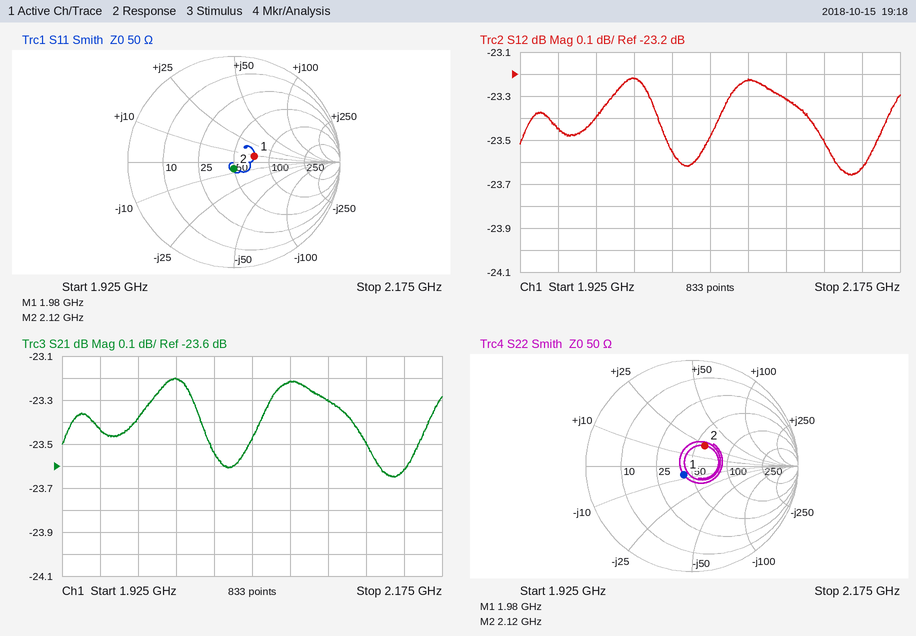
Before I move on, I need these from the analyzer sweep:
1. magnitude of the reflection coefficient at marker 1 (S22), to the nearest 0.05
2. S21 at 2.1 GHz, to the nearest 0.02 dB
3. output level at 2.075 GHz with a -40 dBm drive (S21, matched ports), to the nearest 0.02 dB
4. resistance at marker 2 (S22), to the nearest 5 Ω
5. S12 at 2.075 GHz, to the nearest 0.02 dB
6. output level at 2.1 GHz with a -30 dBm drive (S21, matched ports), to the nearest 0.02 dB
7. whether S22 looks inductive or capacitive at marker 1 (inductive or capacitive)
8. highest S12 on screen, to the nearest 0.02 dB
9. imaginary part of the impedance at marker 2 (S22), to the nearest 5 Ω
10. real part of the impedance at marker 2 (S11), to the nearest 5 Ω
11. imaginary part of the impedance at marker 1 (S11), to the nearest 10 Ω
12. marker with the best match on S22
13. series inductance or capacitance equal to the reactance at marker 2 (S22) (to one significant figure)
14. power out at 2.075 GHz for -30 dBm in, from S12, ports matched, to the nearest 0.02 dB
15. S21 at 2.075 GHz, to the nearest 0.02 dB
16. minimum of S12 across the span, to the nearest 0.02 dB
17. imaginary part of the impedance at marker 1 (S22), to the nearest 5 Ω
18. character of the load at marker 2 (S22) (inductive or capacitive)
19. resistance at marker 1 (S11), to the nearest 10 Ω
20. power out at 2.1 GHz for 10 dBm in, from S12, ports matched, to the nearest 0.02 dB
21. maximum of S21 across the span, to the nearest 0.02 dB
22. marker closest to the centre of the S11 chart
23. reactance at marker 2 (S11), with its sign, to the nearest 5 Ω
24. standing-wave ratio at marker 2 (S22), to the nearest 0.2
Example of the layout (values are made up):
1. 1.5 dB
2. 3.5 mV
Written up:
1. 0.10
2. -23.30 dB
3. -63.22 dBm
4. 60 Ω
5. -23.22 dB
6. -53.30 dBm
7. capacitive
8. -23.22 dB
9. +25 Ω
10. 50 Ω
11. +10 Ω
12. marker 1
13. 2 nH
14. -53.22 dBm
15. -23.22 dB
16. -23.66 dB
17. -5 Ω
18. inductive
19. 70 Ω
20. -13.32 dBm
21. -23.20 dB
22. marker 2
23. -5 Ω
24. 1.6
